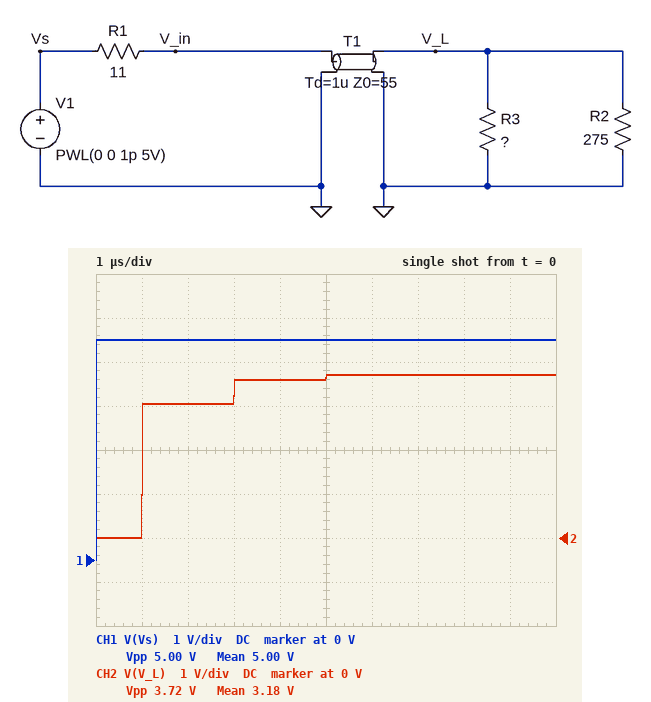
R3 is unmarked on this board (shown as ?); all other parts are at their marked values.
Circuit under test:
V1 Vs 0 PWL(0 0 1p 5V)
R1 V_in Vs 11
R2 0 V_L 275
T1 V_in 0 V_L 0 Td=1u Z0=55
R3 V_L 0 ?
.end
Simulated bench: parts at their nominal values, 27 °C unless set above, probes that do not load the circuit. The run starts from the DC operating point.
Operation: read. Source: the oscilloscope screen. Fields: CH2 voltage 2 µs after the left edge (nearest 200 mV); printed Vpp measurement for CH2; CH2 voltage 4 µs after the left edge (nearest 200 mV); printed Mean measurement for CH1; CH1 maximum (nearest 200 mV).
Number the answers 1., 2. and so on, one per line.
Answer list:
1. 3.0 V
2. 3.72 V
3. 3.6 V
4. 5.00 V
5. 5.0 V
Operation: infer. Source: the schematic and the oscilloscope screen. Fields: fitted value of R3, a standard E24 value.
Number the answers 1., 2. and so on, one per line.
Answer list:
1. 36 Ω
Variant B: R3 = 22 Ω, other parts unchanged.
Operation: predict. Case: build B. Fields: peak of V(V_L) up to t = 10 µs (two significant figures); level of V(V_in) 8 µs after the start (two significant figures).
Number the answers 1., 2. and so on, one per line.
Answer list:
1. 3.2 V
2. 3.3 V
